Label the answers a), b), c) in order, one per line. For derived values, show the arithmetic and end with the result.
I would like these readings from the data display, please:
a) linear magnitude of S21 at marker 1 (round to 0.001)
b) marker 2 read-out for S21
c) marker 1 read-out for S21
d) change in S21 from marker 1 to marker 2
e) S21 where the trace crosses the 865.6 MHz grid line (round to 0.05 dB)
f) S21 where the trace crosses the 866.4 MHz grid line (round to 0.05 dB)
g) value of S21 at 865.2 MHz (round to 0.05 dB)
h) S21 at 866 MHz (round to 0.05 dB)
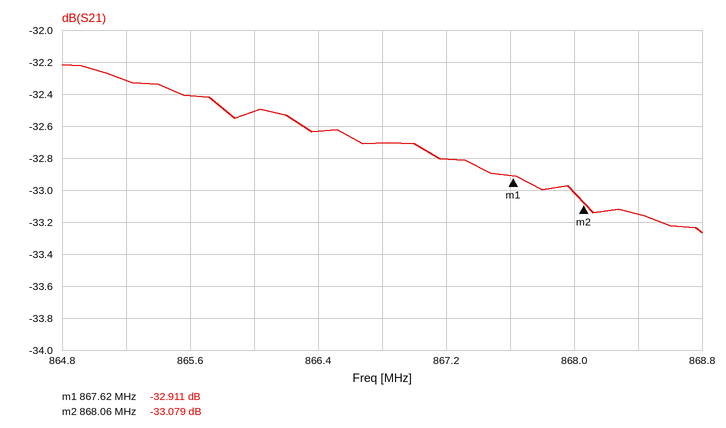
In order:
a) 10^(-32.911/20) ≈ 0.023
b) -33.079 dB
c) -32.911 dB
d) -33.079 − (-32.911) = -0.168 dB
e) -32.40 dB
f) -32.65 dB
g) -32.30 dB
h) -32.50 dB
